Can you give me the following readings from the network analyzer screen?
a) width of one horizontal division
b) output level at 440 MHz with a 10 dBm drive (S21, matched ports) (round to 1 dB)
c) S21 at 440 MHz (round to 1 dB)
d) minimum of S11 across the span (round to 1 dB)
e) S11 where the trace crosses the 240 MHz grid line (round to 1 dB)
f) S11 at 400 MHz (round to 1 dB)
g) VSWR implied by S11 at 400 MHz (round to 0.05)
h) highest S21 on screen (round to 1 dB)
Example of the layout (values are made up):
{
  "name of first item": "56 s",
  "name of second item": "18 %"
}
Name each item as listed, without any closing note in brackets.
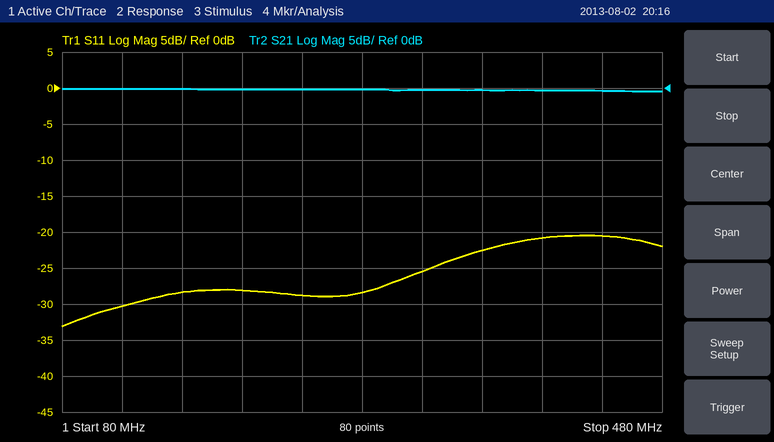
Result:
{
  "width of one horizontal division": "40 MHz",
  "output level at 440 MHz with a 10 dBm drive (S21, matched ports)": "10 dBm",
  "S21 at 440 MHz": "0 dB",
  "minimum of S11 across the span": "-33 dB",
  "S11 where the trace crosses the 240 MHz grid line": "-29 dB",
  "S11 at 400 MHz": "-21 dB",
  "VSWR implied by S11 at 400 MHz": "1.20",
  "highest S21 on screen": "0 dB"
}
